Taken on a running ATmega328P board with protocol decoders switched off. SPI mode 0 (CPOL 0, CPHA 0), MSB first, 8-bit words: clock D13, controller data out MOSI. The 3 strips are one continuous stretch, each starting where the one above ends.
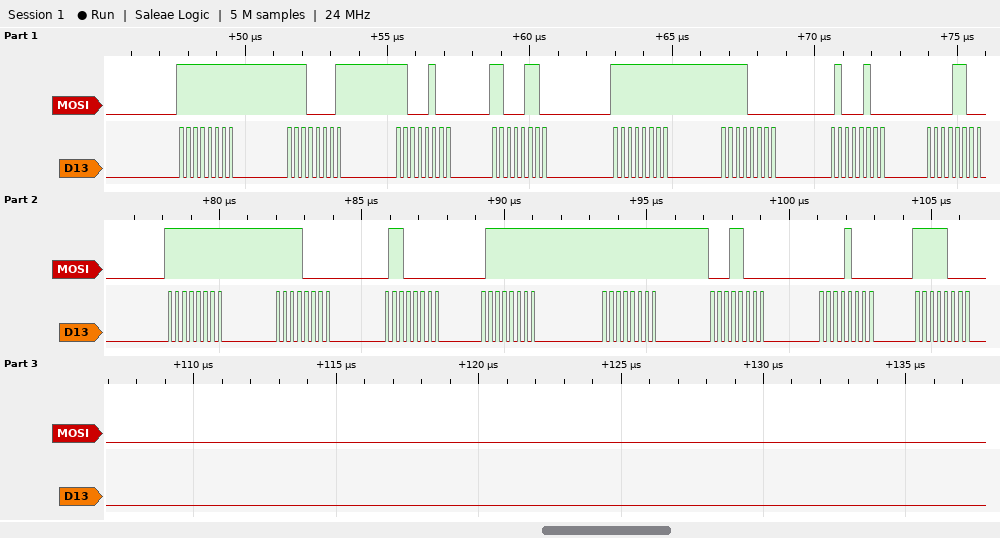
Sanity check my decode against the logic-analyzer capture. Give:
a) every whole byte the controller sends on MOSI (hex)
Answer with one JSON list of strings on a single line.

["FF E1 C4 C6 FF F0 44 0C FF F0 60 7F FF 18 08 F8"]
